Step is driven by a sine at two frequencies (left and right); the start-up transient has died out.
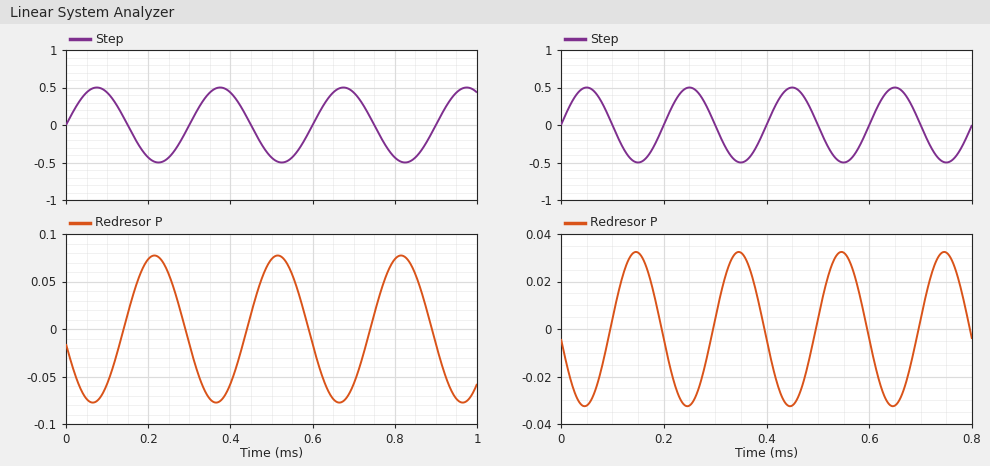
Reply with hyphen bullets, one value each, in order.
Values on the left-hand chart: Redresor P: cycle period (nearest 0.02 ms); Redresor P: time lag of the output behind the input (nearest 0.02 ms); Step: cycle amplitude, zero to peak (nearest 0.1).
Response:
- 0.30 ms
- 0.14 ms
- 0.5
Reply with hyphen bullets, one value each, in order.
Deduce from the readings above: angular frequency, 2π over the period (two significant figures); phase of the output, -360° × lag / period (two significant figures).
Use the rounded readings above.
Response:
- 21 rad/ms
- -170°
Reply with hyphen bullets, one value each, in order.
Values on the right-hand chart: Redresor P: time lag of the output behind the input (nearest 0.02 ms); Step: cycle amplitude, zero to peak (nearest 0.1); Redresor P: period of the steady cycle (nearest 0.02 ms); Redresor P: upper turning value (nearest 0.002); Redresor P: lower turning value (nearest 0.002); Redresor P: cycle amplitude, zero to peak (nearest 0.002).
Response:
- 0.10 ms
- 0.5
- 0.20 ms
- 0.032
- -0.032
- 0.032
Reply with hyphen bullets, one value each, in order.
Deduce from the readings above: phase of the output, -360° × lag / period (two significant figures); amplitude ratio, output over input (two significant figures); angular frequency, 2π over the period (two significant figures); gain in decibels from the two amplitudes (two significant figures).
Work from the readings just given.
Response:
- -180°
- 0.064
- 31 rad/ms
- -24 dB
